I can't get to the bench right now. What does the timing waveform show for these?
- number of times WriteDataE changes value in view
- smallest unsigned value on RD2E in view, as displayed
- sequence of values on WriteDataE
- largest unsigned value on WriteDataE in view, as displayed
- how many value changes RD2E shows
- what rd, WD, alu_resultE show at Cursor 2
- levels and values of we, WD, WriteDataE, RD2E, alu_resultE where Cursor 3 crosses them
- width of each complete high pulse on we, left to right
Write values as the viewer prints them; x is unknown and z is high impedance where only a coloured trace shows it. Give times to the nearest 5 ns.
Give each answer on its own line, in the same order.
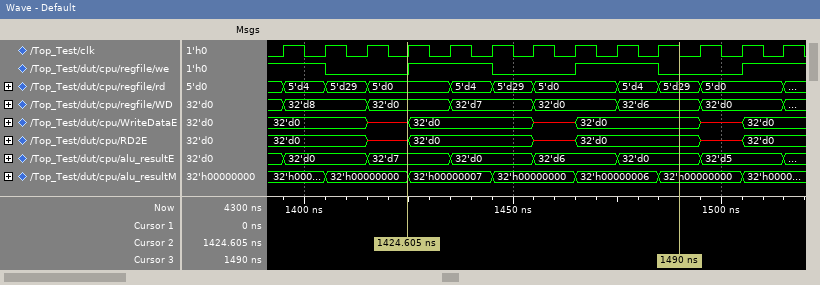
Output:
6
32'd0
32'd0, x, 32'd0, x, 32'd0, x, 32'd0
32'd0
6
rd=5'd0, WD=32'd0, alu_resultE=32'd7
we=0, WD=32'd6, WriteDataE=32'd0, RD2E=32'd0, alu_resultE=32'd0
20 ns, 20 ns
